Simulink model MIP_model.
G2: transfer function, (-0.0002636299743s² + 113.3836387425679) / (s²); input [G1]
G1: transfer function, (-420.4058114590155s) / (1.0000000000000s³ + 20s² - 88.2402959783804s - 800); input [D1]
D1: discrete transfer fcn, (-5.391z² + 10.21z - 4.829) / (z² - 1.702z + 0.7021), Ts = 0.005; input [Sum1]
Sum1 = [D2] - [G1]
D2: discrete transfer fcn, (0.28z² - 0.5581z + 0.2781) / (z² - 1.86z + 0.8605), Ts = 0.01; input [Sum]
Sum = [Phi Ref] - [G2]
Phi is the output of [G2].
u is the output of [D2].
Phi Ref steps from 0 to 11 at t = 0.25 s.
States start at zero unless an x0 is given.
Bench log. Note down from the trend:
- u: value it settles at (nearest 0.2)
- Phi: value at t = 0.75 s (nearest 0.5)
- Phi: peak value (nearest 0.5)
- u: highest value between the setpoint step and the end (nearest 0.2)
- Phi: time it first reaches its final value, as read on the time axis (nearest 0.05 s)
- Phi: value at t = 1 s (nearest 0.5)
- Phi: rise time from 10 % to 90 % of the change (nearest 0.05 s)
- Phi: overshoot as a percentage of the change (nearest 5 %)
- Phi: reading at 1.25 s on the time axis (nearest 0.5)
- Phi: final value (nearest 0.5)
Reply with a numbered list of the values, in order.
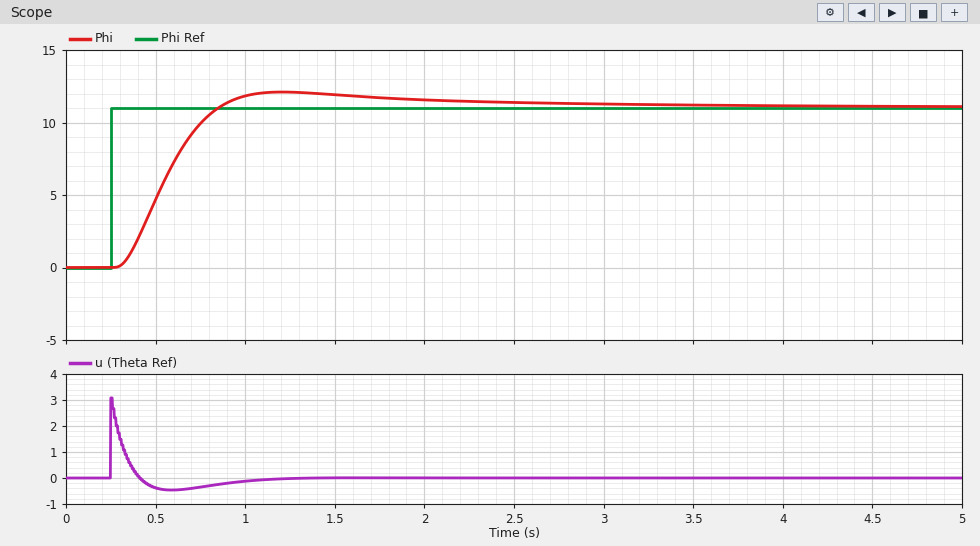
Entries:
1. 0.0
2. 10.0
3. 12.0
4. 3.0
5. 0.85 s
6. 12.0
7. 0.40 s
8. 10 %
9. 12.0
10. 11.0
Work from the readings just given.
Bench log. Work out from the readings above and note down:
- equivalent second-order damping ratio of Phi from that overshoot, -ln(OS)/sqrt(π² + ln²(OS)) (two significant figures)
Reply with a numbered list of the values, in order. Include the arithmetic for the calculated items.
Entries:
1. ln(0.1) = -2.303; 2.303 / sqrt(9.870 + 5.302) = 0.59
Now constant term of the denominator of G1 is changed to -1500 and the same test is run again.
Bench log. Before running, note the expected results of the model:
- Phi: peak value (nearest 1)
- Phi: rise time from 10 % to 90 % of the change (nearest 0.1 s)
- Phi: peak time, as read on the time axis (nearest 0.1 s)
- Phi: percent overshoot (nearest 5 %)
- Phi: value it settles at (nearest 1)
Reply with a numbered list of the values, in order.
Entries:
1. 14
2. 0.3 s
3. 1.1 s
4. 25 %
5. 11
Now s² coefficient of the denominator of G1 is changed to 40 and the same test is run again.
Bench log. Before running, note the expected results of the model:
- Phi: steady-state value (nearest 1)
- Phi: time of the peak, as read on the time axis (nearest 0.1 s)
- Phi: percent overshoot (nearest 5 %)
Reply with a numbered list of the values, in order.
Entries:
1. 11
2. 1.1 s
3. 15 %
